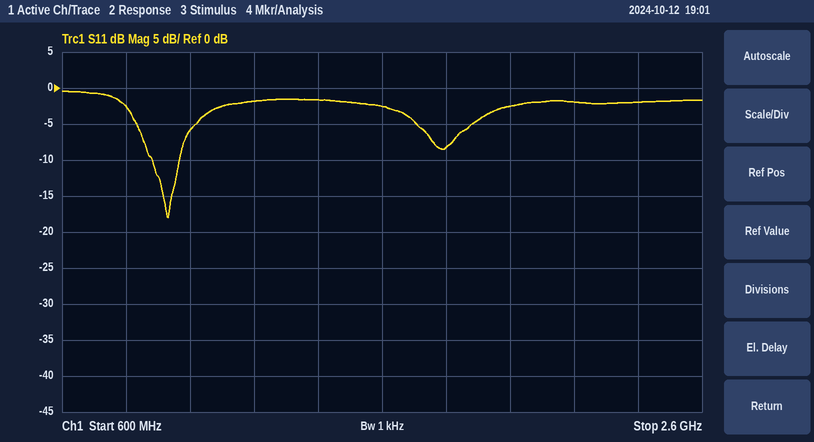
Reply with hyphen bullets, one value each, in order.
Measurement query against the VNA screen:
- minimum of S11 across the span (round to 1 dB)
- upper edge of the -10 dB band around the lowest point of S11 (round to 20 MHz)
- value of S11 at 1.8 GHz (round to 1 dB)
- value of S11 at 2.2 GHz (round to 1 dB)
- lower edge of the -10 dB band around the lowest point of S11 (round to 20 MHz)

- -18 dB
- 960 MHz
- -8 dB
- -2 dB
- 880 MHz
